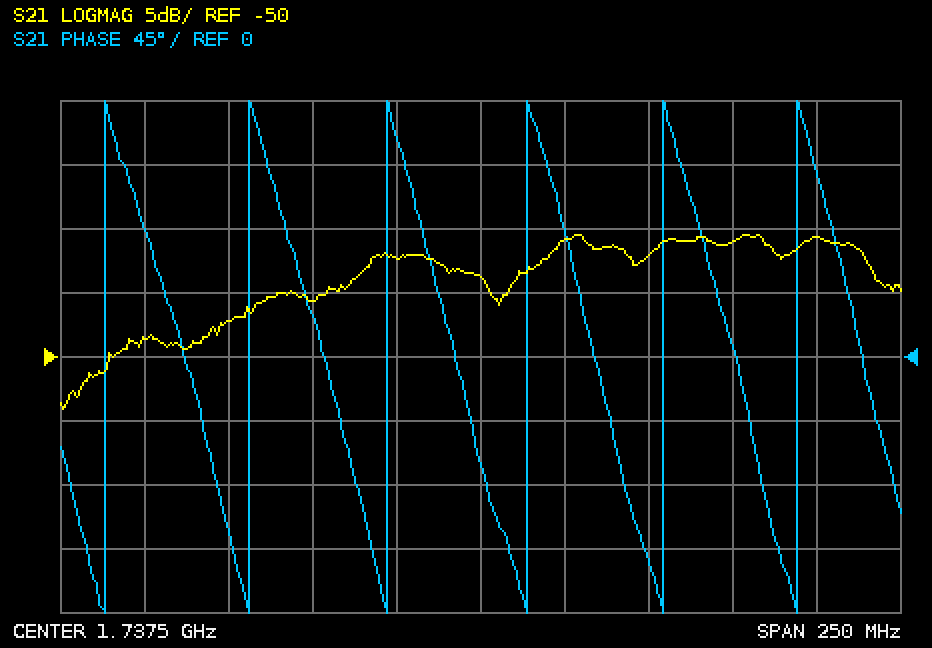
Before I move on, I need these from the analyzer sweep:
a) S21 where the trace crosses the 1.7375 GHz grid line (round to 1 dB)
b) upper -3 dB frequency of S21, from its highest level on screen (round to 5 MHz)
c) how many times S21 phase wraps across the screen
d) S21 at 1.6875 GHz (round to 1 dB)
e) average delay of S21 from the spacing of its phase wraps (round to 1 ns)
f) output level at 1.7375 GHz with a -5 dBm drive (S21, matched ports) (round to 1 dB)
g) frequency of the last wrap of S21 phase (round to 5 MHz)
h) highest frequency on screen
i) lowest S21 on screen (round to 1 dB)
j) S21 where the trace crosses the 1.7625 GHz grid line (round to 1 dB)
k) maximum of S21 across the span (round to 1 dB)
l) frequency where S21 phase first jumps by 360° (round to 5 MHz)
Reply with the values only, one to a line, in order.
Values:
-44 dB
1.855 GHz
6
-46 dB
24 ns
-49 dBm
1.830 GHz
1.8625 GHz
-54 dB
-41 dB
-40 dB
1.625 GHz
